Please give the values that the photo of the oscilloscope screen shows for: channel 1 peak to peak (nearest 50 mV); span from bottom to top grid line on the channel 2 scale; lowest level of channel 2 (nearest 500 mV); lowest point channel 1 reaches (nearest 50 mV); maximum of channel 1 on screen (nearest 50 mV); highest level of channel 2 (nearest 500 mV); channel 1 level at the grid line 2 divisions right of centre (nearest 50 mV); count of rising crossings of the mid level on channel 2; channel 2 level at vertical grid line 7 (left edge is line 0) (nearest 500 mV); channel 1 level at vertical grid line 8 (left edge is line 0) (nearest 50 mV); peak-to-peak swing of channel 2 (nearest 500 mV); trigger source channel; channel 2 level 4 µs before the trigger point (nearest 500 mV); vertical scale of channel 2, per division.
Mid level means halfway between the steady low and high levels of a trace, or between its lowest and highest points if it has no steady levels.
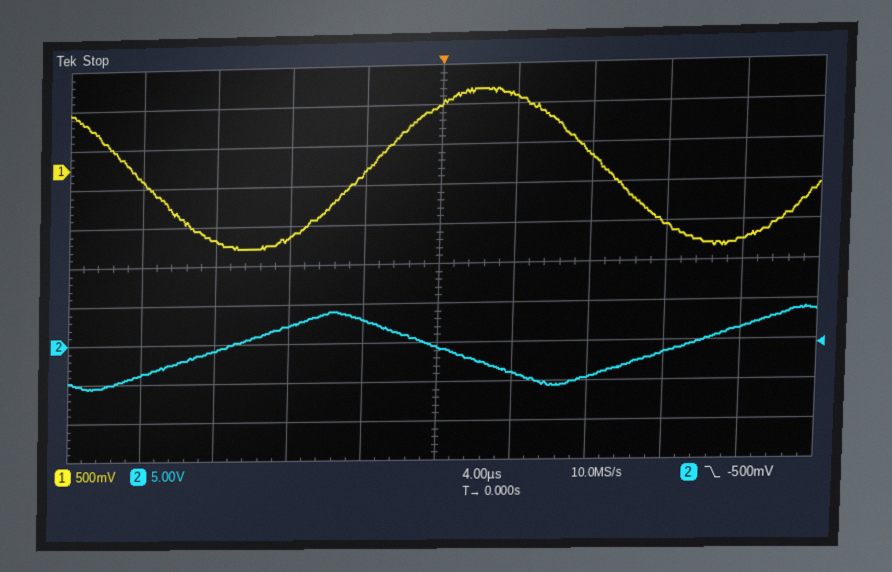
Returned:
2.00 V
50 V
-5.5 V
-1.05 V
950 mV
4.0 V
100 mV
2
-4.5 V
-800 mV
9.5 V
channel 2
3.0 V
5 V
